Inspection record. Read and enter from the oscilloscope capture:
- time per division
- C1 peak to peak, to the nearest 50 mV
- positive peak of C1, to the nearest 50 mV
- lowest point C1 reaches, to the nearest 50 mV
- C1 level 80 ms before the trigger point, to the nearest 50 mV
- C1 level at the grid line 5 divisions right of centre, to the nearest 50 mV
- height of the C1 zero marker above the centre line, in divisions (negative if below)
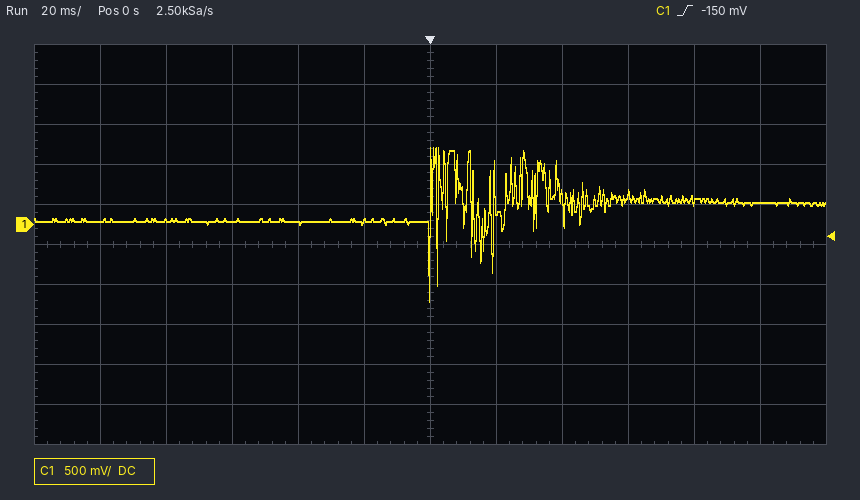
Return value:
20 ms
1.90 V
950 mV
-950 mV
50 mV
300 mV
+0.5 div
